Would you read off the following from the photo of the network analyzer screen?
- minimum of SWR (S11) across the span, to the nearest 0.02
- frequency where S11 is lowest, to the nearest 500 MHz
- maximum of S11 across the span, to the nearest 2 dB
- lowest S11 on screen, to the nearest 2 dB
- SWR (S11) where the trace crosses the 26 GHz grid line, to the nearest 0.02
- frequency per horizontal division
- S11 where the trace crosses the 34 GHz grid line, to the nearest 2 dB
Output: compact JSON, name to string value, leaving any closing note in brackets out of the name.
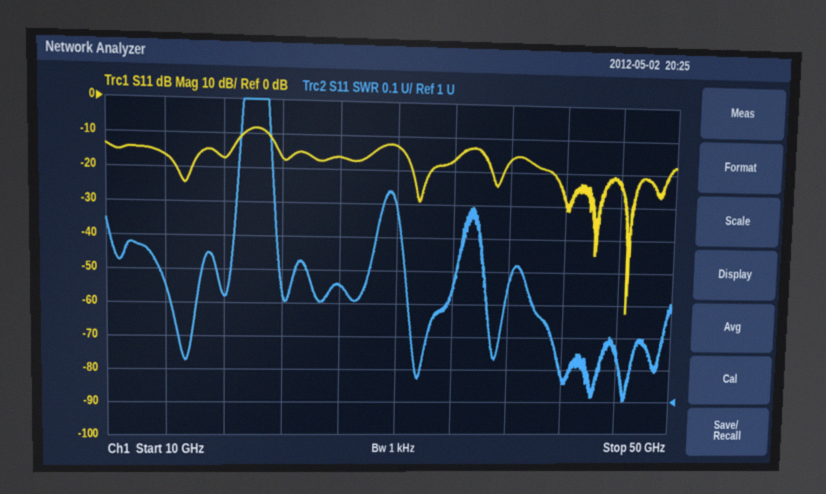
{"minimum of SWR (S11) across the span, to the nearest 0.02": "1.00", "frequency where S11 is lowest, to the nearest 500 MHz": "46.5 GHz", "maximum of S11 across the span, to the nearest 2 dB": "-8 dB", "lowest S11 on screen, to the nearest 2 dB": "-62 dB", "SWR (S11) where the trace crosses the 26 GHz grid line, to the nearest 0.02": "1.36", "frequency per horizontal division": "4 GHz", "S11 where the trace crosses the 34 GHz grid line, to the nearest 2 dB": "-16 dB"}
